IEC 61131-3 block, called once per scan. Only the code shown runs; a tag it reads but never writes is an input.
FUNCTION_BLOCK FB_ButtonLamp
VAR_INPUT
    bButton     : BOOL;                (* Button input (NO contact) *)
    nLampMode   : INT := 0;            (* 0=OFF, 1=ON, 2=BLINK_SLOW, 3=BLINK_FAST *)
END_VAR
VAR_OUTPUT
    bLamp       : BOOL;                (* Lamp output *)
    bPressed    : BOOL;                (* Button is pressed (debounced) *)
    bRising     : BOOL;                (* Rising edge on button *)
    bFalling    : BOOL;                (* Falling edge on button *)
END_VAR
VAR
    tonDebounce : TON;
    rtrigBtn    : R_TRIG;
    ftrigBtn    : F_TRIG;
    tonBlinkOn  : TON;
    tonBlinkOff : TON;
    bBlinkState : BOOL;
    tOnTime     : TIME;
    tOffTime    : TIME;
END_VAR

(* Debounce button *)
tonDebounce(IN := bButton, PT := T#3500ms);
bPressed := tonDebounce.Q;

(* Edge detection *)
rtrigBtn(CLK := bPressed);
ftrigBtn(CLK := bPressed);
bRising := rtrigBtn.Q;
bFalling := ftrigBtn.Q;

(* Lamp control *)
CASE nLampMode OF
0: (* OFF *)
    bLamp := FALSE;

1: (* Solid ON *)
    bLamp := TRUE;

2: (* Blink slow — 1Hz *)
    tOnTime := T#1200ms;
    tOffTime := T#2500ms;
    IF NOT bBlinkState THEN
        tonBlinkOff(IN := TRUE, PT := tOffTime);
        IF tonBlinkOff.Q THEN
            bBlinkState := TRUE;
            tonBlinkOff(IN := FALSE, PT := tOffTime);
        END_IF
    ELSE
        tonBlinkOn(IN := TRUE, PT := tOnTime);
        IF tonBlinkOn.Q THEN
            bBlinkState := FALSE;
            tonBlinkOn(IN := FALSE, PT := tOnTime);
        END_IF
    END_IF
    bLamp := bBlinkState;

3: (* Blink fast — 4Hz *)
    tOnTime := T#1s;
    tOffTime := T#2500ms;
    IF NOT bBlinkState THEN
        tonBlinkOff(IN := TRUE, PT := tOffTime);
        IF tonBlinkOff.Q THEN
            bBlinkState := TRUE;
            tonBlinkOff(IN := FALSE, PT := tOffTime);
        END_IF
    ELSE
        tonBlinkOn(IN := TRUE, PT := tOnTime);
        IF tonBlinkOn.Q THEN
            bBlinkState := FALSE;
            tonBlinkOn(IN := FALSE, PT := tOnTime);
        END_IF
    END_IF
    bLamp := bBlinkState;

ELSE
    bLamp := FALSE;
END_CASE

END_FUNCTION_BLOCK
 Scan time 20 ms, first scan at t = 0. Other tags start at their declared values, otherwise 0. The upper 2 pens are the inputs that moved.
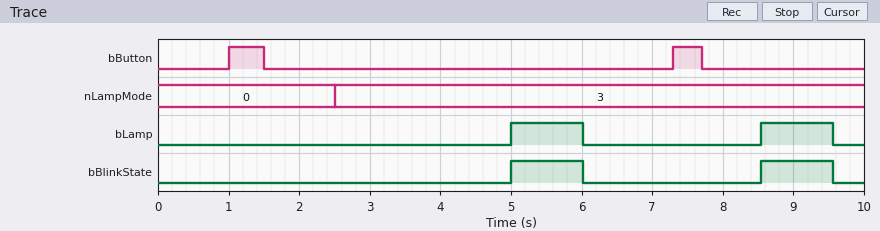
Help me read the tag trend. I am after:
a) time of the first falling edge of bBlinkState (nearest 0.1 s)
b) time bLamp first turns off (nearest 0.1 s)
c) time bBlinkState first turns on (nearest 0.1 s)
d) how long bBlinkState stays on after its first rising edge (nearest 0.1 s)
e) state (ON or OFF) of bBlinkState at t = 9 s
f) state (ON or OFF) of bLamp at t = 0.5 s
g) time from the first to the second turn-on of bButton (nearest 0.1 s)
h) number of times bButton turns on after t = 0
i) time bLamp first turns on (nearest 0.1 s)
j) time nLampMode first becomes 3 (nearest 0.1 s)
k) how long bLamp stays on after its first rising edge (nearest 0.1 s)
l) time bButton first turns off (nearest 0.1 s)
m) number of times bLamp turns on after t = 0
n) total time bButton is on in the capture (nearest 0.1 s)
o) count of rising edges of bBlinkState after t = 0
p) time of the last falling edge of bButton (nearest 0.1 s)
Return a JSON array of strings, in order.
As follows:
["6.0 s", "6.0 s", "5.0 s", "1.0 s", "ON", "OFF", "6.3 s", "2", "5.0 s", "2.5 s", "1.0 s", "1.5 s", "2", "0.9 s", "2", "7.7 s"]
